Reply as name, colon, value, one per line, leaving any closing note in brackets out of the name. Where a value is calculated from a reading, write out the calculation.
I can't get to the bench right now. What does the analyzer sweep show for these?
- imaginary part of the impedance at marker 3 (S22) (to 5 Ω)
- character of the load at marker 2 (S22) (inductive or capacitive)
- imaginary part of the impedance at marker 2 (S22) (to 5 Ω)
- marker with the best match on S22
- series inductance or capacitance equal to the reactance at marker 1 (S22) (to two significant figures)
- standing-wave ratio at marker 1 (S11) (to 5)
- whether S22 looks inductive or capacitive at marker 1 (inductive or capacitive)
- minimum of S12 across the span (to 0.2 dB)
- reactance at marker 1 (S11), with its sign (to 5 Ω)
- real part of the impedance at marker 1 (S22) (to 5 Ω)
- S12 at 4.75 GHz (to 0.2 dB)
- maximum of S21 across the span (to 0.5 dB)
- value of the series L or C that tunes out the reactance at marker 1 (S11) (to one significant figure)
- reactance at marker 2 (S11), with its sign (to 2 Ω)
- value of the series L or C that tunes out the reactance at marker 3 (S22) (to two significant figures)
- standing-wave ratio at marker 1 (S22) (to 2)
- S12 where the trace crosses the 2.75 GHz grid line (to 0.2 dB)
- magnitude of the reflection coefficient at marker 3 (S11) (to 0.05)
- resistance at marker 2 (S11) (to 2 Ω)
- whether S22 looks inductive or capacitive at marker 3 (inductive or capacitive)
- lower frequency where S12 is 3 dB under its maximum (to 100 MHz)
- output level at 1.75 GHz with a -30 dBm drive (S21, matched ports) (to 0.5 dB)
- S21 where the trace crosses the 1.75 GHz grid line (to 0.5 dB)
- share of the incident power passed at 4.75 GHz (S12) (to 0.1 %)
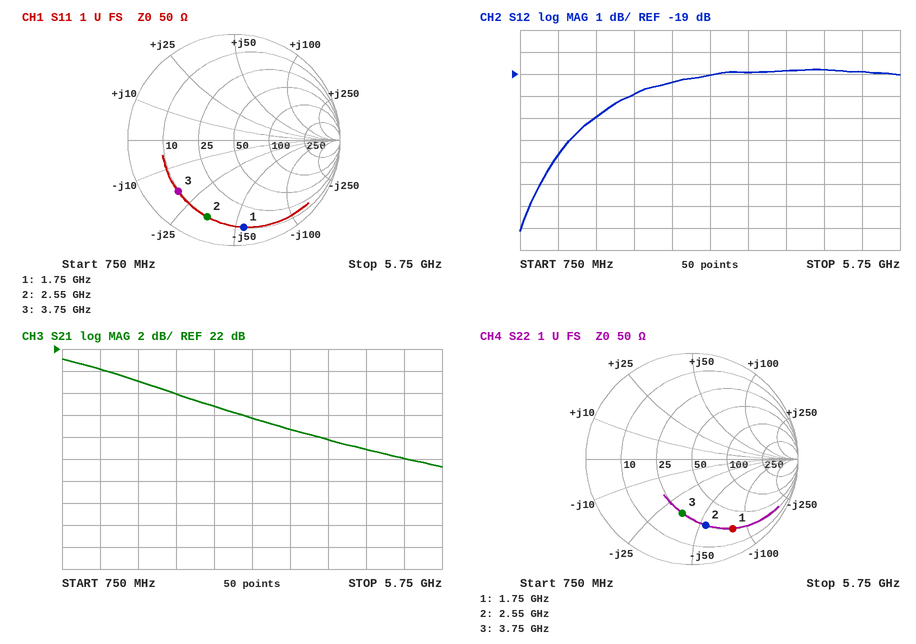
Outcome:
imaginary part of the impedance at marker 3 (S22): -35 Ω
character of the load at marker 2 (S22): capacitive
imaginary part of the impedance at marker 2 (S22): -55 Ω
marker with the best match on S22: marker 3
series inductance or capacitance equal to the reactance at marker 1 (S22): C = 1/(2π × 1.75 GHz × 80 Ω) ≈ 1.1 pF
standing-wave ratio at marker 1 (S11): 10
whether S22 looks inductive or capacitive at marker 1: capacitive
minimum of S12 across the span: -26.2 dB
reactance at marker 1 (S11), with its sign: -55 Ω
real part of the impedance at marker 1 (S22): 25 Ω
S12 at 4.75 GHz: -18.8 dB
maximum of S21 across the span: 21.0 dB
value of the series L or C that tunes out the reactance at marker 1 (S11): L = 55 Ω/(2π × 1.75 GHz) ≈ 5 nH
reactance at marker 2 (S11), with its sign: -34 Ω
value of the series L or C that tunes out the reactance at marker 3 (S22): L = 35 Ω/(2π × 3.75 GHz) ≈ 1.5 nH
standing-wave ratio at marker 1 (S22): 8
S12 where the trace crosses the 2.75 GHz grid line: -19.4 dB
magnitude of the reflection coefficient at marker 3 (S11): 0.70
resistance at marker 2 (S11): 10 Ω
whether S22 looks inductive or capacitive at marker 3: capacitive
lower frequency where S12 is 3 dB under its maximum: 1.5 GHz
output level at 1.75 GHz with a -30 dBm drive (S21, matched ports): -30 dBm + (19.0 dB) = -11.0 dBm
S21 where the trace crosses the 1.75 GHz grid line: 19.0 dB
share of the incident power passed at 4.75 GHz (S12): 10^(-18.8/10) ≈ 1.3 %
